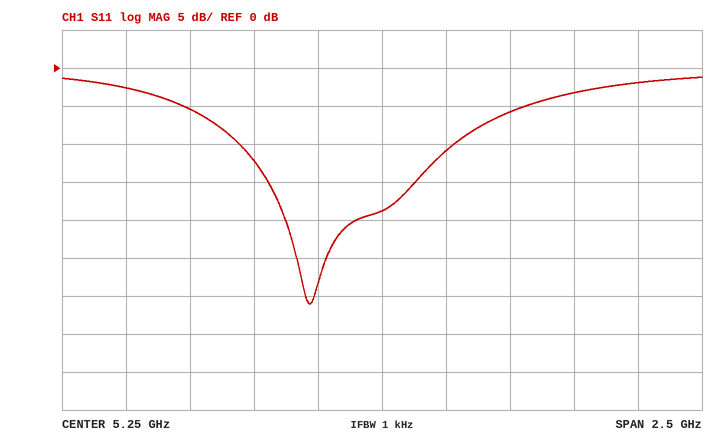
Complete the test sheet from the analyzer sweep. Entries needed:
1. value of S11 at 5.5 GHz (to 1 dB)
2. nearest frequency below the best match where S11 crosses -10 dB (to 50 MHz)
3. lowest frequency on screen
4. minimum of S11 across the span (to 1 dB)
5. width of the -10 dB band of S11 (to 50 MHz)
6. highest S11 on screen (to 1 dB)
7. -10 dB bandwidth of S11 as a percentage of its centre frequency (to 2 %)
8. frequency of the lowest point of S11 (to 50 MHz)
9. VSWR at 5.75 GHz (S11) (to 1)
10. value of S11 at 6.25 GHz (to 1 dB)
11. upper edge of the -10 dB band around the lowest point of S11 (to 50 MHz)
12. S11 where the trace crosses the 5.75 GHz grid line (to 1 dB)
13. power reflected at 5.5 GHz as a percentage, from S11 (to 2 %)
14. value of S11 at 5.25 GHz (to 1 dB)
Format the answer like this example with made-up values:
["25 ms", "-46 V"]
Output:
["-11 dB", "4.70 GHz", "4 GHz", "-31 dB", "850 MHz", "-1 dB", "16 %", "4.95 GHz", "3", "-2 dB", "5.55 GHz", "-6 dB", "8 %", "-19 dB"]
